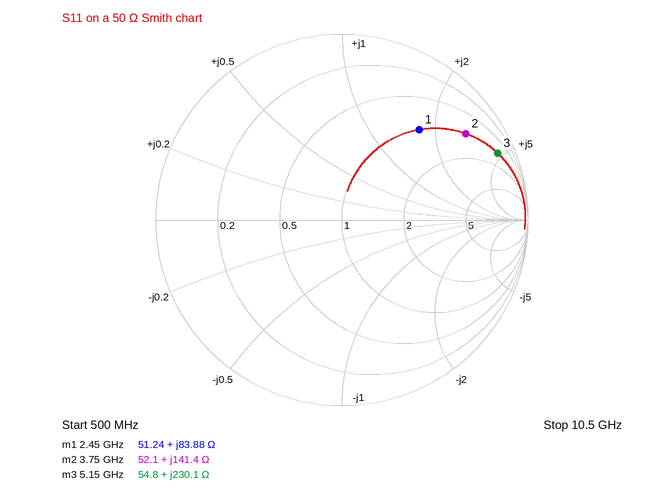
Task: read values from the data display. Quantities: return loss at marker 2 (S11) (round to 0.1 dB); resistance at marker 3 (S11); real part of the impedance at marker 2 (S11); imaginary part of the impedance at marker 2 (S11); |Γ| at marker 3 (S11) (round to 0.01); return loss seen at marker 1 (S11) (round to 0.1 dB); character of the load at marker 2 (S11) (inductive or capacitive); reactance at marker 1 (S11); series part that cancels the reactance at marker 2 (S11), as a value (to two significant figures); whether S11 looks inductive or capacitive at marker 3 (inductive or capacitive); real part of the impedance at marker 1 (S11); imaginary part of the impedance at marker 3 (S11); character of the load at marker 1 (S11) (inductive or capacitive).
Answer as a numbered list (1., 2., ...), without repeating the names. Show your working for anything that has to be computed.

1. 1.8 dB
2. 54.8 Ω
3. 52.1 Ω
4. +141.4 Ω
5. 0.91
6. 3.9 dB
7. inductive
8. +83.88 Ω
9. C = 1/(2π × 3.75 GHz × 141.4 Ω) ≈ 300 fF
10. inductive
11. 51.24 Ω
12. +230.1 Ω
13. inductive
